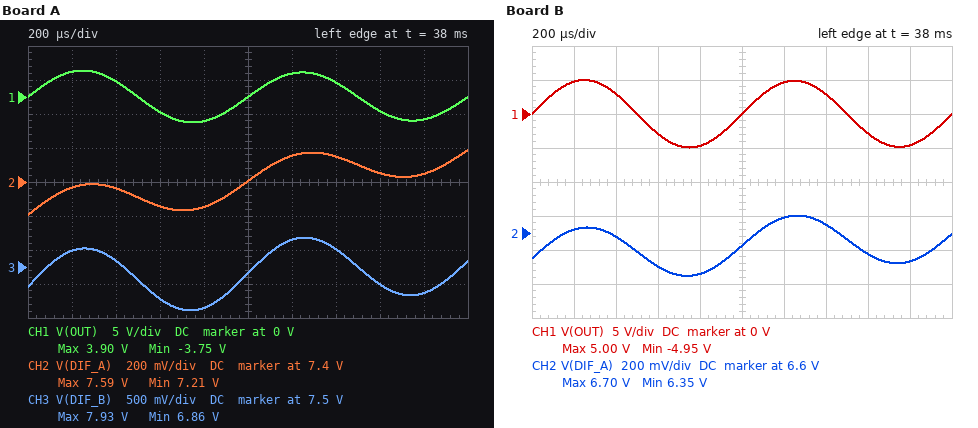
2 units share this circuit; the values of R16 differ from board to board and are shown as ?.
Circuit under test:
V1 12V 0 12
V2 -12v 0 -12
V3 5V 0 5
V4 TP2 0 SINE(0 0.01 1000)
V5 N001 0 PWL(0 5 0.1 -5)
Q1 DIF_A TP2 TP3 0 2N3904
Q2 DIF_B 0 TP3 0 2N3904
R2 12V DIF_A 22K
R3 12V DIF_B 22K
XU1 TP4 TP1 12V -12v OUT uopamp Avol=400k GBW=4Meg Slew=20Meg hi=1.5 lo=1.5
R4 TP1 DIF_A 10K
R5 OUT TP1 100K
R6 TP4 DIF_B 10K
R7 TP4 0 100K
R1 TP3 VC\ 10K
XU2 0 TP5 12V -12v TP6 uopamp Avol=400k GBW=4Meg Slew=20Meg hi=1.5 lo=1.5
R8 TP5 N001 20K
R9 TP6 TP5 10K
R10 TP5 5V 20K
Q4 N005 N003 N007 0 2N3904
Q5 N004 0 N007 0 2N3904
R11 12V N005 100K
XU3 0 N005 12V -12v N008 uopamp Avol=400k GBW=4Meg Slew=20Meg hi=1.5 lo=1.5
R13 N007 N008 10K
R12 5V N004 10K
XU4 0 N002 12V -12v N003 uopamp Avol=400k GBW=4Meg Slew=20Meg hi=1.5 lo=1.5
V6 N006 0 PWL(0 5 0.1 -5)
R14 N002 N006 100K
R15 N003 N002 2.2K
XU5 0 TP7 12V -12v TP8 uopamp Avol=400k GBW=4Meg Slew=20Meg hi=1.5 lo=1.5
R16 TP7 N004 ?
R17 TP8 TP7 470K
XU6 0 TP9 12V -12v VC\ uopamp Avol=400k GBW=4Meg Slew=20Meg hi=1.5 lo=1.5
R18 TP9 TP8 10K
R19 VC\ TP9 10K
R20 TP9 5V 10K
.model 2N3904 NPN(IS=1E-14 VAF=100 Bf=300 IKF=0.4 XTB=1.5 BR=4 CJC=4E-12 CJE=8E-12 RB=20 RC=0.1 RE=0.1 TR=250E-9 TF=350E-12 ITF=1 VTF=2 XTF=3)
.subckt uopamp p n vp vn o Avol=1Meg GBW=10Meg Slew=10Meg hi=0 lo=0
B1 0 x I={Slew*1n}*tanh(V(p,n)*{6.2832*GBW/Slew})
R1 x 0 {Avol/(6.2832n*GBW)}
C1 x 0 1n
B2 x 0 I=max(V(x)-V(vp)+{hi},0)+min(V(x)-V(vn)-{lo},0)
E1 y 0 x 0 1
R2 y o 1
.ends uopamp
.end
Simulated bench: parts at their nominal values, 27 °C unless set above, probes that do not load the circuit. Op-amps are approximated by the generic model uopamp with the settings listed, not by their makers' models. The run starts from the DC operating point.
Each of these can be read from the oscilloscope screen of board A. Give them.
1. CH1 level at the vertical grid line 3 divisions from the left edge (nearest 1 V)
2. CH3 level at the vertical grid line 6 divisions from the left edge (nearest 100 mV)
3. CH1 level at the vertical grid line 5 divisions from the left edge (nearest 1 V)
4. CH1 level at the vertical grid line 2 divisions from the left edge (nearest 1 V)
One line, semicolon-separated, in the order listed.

-2 V; 7.9 V; 0 V; 2 V
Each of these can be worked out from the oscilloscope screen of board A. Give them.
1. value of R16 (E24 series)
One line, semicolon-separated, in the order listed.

560 kΩ
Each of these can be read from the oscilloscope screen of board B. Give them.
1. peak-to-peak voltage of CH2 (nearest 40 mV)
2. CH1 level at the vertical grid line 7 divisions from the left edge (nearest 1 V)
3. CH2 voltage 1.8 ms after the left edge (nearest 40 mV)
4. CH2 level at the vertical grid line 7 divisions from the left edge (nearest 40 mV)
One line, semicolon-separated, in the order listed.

360 mV; 3 V; 6.44 V; 6.64 V
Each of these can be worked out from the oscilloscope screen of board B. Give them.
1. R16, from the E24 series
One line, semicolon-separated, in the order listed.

1.5 MΩ
